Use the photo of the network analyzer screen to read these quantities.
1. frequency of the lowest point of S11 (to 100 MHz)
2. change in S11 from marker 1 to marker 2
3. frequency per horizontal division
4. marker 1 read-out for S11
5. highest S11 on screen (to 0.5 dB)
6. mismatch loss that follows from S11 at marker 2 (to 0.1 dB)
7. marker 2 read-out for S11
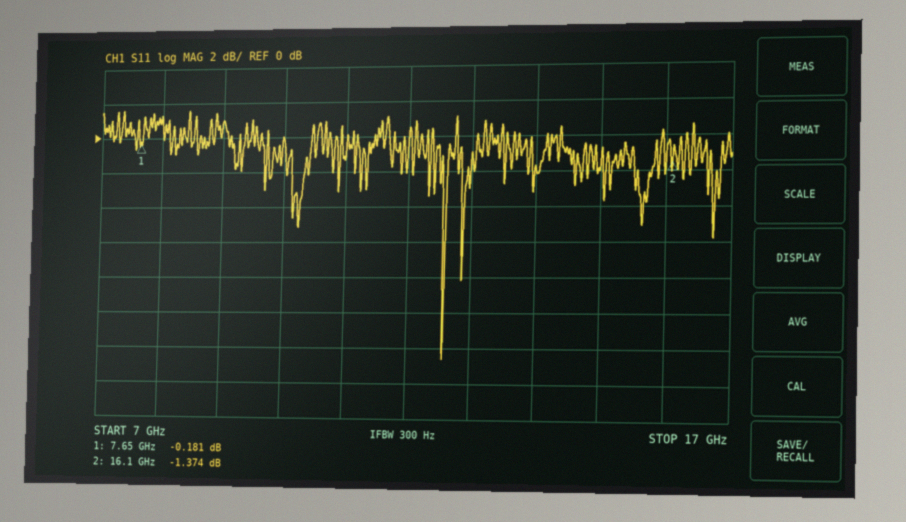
12.6 GHz
-1.193 dB
1 GHz
-0.181 dB
1.5 dB
5.7 dB
-1.374 dB
